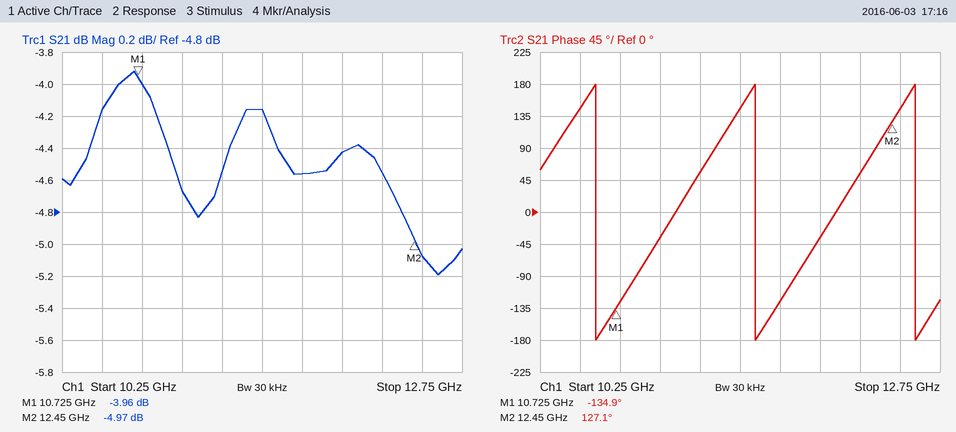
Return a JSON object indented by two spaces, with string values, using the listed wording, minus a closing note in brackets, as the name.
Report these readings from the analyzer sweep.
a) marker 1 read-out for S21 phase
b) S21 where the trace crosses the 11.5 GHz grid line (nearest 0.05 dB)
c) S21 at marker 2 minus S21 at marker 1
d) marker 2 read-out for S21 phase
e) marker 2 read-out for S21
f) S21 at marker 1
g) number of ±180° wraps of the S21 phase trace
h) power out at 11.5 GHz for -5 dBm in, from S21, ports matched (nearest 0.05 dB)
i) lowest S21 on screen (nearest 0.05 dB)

{
  "marker 1 read-out for S21 phase": "-134.9°",
  "S21 where the trace crosses the 11.5 GHz grid line": "-4.15 dB",
  "S21 at marker 2 minus S21 at marker 1": "-1.01 dB",
  "marker 2 read-out for S21 phase": "127.1°",
  "marker 2 read-out for S21": "-4.97 dB",
  "S21 at marker 1": "-3.96 dB",
  "number of ±180° wraps of the S21 phase trace": "3",
  "power out at 11.5 GHz for -5 dBm in, from S21, ports matched": "-9.15 dBm",
  "lowest S21 on screen": "-5.20 dB"
}
